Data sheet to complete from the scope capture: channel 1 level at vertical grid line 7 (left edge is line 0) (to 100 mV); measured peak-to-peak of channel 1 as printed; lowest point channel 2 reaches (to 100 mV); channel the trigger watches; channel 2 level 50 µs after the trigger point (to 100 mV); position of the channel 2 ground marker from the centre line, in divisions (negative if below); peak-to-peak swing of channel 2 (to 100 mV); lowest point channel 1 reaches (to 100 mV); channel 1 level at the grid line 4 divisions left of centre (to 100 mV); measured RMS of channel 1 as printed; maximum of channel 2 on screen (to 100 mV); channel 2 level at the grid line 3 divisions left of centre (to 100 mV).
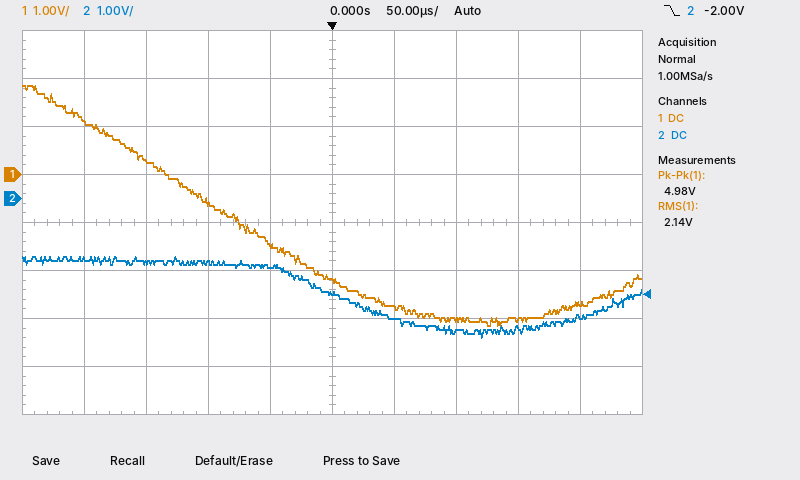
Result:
-3.0 V
4.98 V
-2.9 V
channel 2
-2.5 V
+0.5 div
1.7 V
-3.1 V
1.1 V
2.14 V
-1.2 V
-1.3 V
